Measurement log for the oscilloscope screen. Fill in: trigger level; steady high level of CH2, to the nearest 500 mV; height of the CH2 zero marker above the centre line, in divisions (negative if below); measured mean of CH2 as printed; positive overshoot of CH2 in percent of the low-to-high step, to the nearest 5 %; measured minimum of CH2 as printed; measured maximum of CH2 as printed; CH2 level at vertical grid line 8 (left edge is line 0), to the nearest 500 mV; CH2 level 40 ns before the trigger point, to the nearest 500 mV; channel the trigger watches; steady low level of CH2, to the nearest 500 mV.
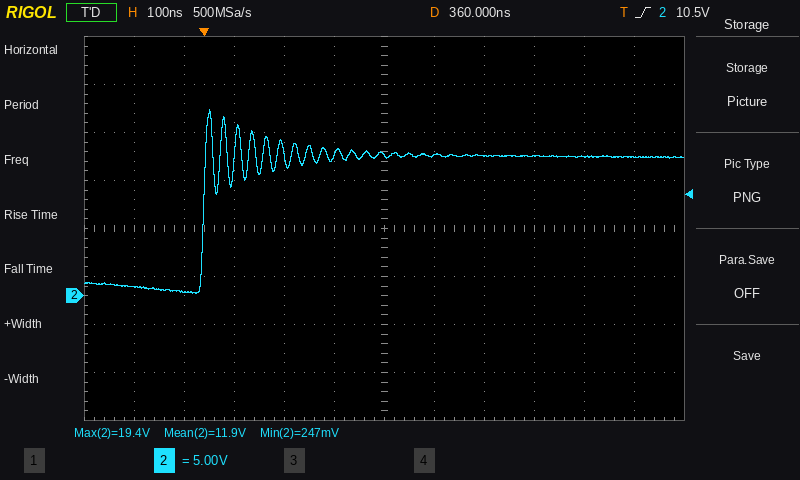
10.5 V
14.5 V
-1.4 div
11.9 V
35 %
247 mV
19.4 V
14.5 V
500 mV
CH2
1.0 V
